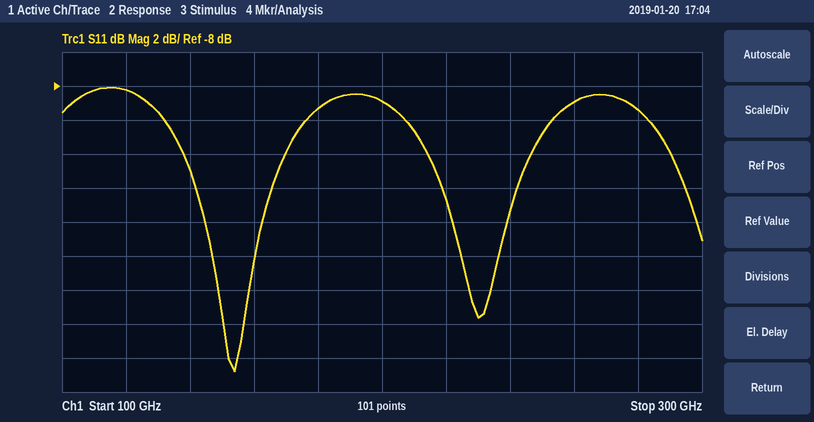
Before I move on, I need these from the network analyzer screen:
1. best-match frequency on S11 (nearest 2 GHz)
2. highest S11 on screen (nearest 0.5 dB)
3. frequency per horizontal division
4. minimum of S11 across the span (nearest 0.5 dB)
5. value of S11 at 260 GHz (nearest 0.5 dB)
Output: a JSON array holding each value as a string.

["154 GHz", "-8.0 dB", "20 GHz", "-25.0 dB", "-9.0 dB"]
